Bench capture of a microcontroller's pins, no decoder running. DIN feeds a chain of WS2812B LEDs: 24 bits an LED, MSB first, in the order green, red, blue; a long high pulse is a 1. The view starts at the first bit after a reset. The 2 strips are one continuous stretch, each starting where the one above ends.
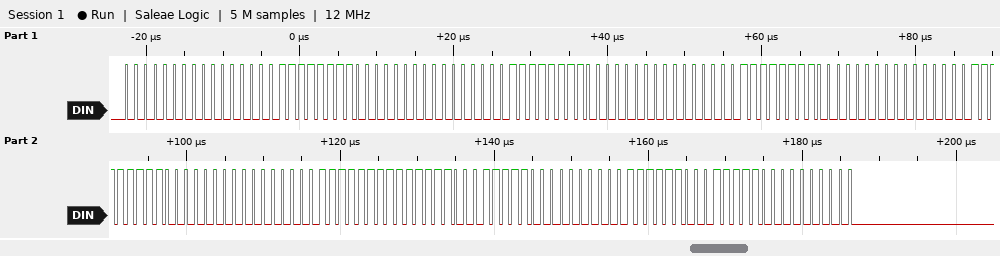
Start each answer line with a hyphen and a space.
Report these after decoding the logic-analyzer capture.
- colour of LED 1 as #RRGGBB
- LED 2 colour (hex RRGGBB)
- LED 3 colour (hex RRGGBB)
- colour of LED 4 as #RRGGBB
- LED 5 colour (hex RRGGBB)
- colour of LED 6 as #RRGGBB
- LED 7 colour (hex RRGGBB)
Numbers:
- #0000FF
- #0000FF
- #0000FF
- #0000FF
- #0000FF
- #7CFC00
- #7CFC00
